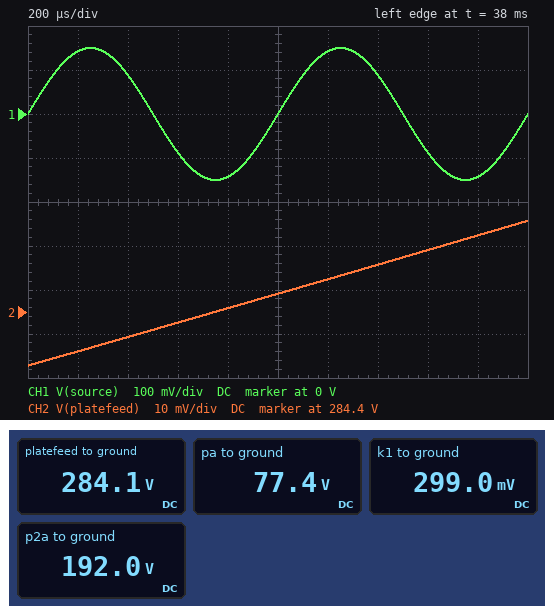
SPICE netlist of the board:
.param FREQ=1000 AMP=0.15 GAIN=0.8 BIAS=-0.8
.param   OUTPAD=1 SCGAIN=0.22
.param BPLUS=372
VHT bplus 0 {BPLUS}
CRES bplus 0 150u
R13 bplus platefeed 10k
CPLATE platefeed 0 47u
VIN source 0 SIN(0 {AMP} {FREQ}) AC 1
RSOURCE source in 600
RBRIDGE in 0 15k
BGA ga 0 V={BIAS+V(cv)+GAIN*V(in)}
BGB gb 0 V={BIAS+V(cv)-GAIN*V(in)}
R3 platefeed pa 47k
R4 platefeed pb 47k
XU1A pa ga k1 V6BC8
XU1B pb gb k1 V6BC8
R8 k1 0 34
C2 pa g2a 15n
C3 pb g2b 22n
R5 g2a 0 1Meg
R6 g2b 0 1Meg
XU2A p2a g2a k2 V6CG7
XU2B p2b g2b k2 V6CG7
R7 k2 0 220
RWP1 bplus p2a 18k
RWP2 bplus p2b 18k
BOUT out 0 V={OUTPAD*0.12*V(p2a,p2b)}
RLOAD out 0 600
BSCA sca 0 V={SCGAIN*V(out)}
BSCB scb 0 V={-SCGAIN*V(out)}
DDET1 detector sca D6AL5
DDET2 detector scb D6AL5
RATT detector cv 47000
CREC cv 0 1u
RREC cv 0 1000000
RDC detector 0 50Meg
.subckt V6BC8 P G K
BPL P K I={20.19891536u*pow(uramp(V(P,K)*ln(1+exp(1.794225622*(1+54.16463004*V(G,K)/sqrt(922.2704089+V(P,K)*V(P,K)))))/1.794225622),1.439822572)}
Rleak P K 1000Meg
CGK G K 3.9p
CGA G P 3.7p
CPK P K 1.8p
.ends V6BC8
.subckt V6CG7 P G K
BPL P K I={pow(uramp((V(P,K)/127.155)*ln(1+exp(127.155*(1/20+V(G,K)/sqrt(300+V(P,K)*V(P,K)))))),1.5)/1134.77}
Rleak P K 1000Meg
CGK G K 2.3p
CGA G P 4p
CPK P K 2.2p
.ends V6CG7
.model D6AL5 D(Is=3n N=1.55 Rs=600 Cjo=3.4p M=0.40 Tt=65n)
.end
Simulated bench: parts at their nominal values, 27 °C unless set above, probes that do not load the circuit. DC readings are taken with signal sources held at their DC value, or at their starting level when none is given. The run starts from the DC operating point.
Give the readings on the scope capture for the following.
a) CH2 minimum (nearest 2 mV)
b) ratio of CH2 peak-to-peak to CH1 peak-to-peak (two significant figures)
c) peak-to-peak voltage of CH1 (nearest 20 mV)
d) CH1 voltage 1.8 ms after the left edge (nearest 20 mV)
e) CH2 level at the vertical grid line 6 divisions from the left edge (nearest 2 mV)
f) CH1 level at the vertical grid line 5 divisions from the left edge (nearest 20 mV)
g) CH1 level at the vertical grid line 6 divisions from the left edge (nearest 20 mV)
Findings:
284.428 V
0.11
300 mV
-140 mV
284.448 V
0 V
140 mV
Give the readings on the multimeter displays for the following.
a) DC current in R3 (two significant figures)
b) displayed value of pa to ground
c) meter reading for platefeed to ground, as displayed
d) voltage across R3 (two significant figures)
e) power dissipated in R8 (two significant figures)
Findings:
4.4 mA
77.4 V
284.1 V
210 V
2.6 mW
